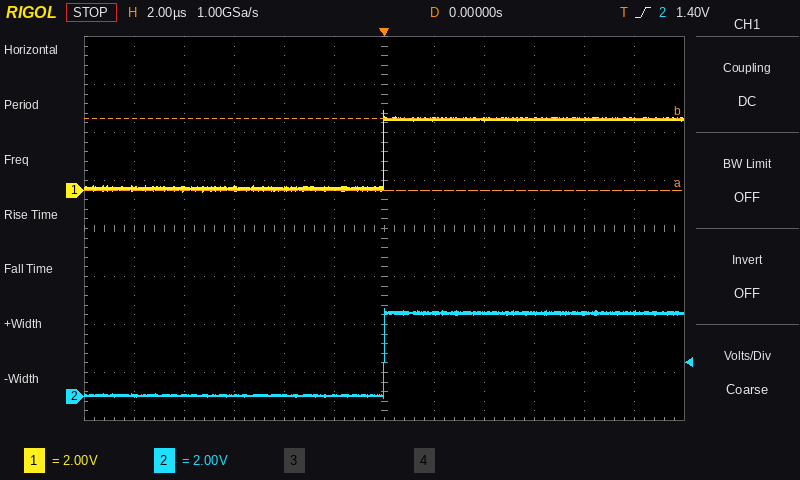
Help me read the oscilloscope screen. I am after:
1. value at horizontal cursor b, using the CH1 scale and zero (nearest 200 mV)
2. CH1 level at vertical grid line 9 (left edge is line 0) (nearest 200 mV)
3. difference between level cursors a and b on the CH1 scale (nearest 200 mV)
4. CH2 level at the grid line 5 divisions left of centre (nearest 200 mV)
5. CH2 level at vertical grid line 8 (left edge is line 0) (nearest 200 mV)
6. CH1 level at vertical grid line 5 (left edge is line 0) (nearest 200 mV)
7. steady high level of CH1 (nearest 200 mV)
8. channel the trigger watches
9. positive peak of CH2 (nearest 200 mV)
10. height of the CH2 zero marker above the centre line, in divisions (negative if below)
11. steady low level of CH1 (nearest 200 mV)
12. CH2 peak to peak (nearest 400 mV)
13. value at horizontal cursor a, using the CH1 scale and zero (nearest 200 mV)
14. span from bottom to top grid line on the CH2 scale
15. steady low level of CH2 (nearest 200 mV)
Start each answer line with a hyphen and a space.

- 3.0 V
- 3.0 V
- 3.0 V
- 0.0 V
- 3.4 V
- 0.0 V
- 3.0 V
- CH2
- 3.6 V
- -3.5 div
- 0.0 V
- 3.6 V
- 0.0 V
- 16 V
- 0.0 V
